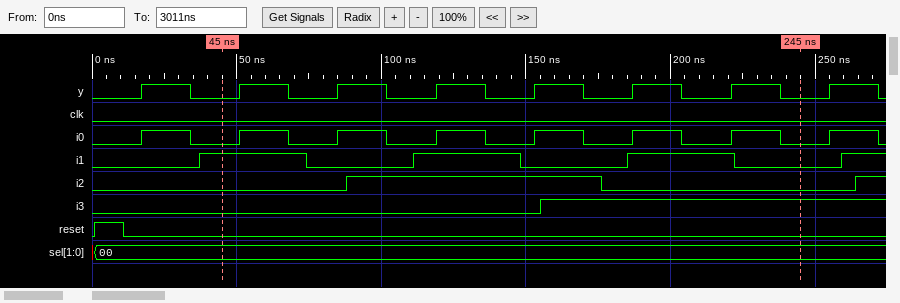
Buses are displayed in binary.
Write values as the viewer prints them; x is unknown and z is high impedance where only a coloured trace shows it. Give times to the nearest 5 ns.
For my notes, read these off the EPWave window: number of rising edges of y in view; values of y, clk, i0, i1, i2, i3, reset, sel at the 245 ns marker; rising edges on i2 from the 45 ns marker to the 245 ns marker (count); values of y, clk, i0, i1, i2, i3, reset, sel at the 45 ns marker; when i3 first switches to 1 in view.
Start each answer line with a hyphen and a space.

- 8
- y=0, clk=0, i0=0, i1=0, i2=0, i3=1, reset=0, sel=00
- 1
- y=0, clk=0, i0=0, i1=1, i2=0, i3=0, reset=0, sel=00
- 155 ns
